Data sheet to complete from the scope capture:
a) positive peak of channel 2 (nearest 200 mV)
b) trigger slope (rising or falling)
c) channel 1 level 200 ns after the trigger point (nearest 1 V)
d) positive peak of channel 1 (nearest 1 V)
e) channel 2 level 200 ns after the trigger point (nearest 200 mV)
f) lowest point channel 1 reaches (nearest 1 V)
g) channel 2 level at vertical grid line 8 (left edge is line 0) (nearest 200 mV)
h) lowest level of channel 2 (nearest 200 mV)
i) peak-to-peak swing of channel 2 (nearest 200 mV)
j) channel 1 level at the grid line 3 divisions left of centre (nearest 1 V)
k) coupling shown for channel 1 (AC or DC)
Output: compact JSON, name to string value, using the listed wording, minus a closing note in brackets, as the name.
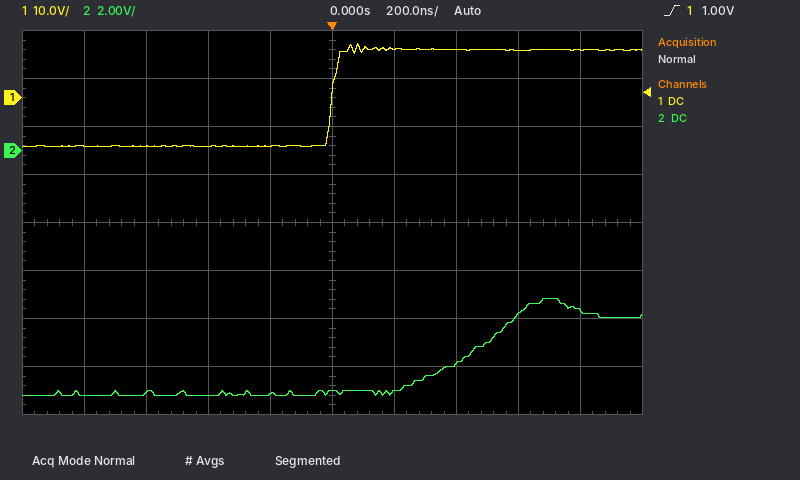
{"positive peak of channel 2": "-6.2 V", "trigger slope": "rising", "channel 1 level 200 ns after the trigger point": "10 V", "positive peak of channel 1": "11 V", "channel 2 level 200 ns after the trigger point": "-10.0 V", "lowest point channel 1 reaches": "-10 V", "channel 2 level at vertical grid line 8 (left edge is line 0)": "-6.8 V", "lowest level of channel 2": "-10.2 V", "peak-to-peak swing of channel 2": "4.0 V", "channel 1 level at the grid line 3 divisions left of centre": "-10 V", "coupling shown for channel 1": "DC"}
